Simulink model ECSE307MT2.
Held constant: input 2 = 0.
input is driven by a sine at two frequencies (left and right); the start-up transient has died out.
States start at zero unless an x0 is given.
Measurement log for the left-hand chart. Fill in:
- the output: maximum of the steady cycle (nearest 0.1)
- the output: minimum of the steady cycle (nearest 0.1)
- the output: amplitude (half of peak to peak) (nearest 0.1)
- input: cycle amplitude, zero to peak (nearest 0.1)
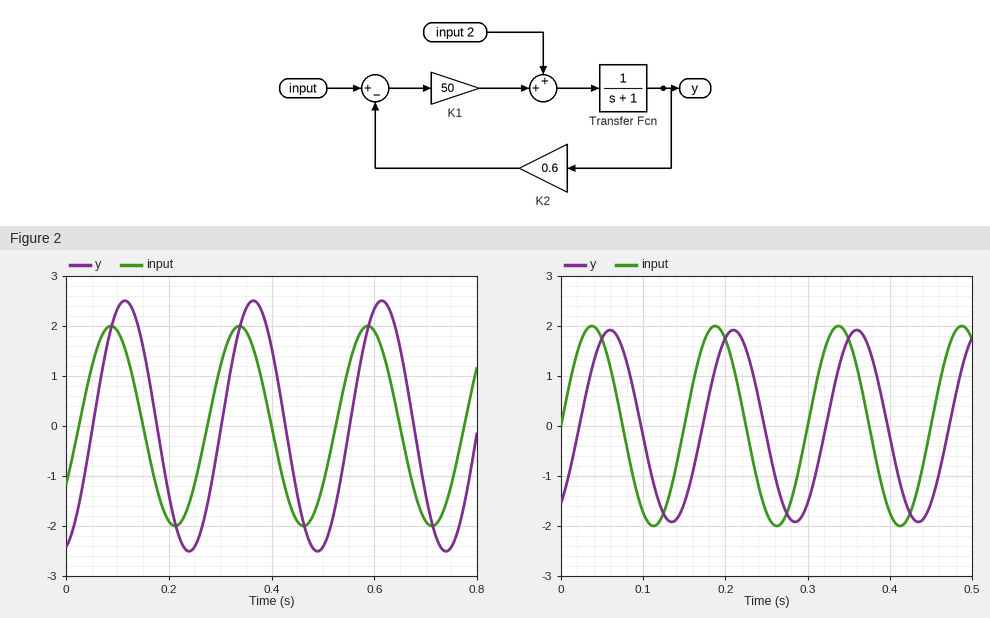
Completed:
2.5
-2.5
2.5
2.0
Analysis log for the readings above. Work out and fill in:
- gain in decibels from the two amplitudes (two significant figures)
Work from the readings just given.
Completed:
1.9 dB
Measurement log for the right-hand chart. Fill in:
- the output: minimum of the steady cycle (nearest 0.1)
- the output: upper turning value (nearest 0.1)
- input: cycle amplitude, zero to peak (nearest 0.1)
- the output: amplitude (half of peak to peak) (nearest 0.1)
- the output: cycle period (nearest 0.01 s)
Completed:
-1.9
1.9
2.0
1.9
0.15 s
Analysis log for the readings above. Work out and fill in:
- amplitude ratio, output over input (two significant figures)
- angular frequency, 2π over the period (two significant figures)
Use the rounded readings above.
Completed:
0.95
42 rad/s
